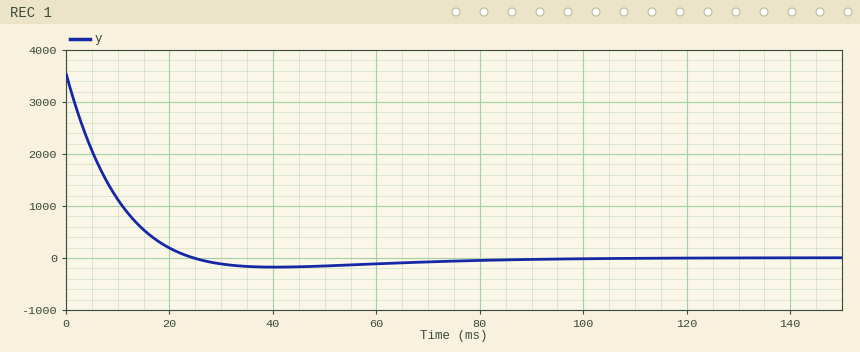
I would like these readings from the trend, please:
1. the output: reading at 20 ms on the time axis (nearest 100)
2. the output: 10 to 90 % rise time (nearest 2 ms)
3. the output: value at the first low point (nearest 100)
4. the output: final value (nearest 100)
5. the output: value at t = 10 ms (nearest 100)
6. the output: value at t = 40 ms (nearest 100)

200
16 ms
-200
0
1100
-200
